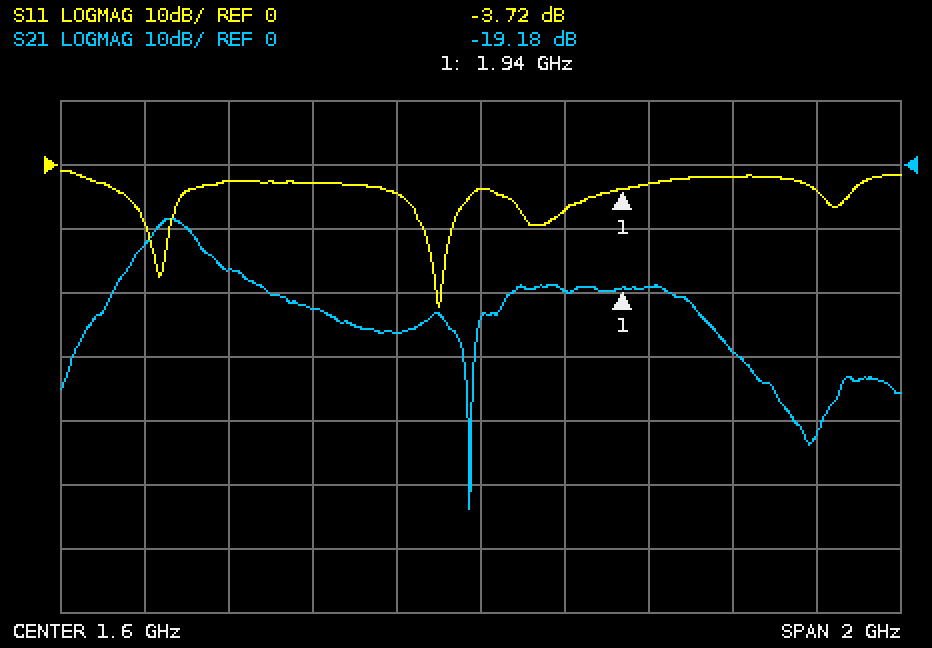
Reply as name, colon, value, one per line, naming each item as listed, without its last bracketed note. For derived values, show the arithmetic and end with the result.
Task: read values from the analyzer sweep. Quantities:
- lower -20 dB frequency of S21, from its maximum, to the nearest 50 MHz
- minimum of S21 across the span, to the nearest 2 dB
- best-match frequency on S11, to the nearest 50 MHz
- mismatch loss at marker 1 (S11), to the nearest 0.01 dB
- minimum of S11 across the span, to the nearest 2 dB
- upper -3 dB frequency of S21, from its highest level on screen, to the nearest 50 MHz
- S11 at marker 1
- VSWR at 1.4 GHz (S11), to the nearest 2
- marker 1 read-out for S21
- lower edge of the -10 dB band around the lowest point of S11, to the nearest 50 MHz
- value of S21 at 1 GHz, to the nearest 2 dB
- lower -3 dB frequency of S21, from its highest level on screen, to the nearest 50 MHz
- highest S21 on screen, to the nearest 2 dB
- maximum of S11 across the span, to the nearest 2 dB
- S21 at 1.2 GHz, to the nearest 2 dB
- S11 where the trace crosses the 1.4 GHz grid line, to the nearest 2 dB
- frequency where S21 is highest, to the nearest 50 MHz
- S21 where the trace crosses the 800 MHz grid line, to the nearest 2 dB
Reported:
lower -20 dB frequency of S21, from its maximum, to the nearest 50 MHz: 650 MHz
minimum of S21 across the span, to the nearest 2 dB: -54 dB
best-match frequency on S11, to the nearest 50 MHz: 1.50 GHz
mismatch loss at marker 1 (S11), to the nearest 0.01 dB: −10 log10(1 − 10^(-3.72/10)) ≈ 2.40 dB
minimum of S11 across the span, to the nearest 2 dB: -22 dB
upper -3 dB frequency of S21, from its highest level on screen, to the nearest 50 MHz: 900 MHz
S11 at marker 1: -3.72 dB
VSWR at 1.4 GHz (S11), to the nearest 2: |Γ| = 10^(-4/20) = 0.6310; VSWR = (1 + 0.6310)/(1 − 0.6310) ≈ 4
marker 1 read-out for S21: -19.18 dB
lower edge of the -10 dB band around the lowest point of S11, to the nearest 50 MHz: 1.45 GHz
value of S21 at 1 GHz, to the nearest 2 dB: -16 dB
lower -3 dB frequency of S21, from its highest level on screen, to the nearest 50 MHz: 800 MHz
highest S21 on screen, to the nearest 2 dB: -8 dB
maximum of S11 across the span, to the nearest 2 dB: 0 dB
S21 at 1.2 GHz, to the nearest 2 dB: -22 dB
S11 where the trace crosses the 1.4 GHz grid line, to the nearest 2 dB: -4 dB
frequency where S21 is highest, to the nearest 50 MHz: 850 MHz
S21 where the trace crosses the 800 MHz grid line, to the nearest 2 dB: -12 dB
